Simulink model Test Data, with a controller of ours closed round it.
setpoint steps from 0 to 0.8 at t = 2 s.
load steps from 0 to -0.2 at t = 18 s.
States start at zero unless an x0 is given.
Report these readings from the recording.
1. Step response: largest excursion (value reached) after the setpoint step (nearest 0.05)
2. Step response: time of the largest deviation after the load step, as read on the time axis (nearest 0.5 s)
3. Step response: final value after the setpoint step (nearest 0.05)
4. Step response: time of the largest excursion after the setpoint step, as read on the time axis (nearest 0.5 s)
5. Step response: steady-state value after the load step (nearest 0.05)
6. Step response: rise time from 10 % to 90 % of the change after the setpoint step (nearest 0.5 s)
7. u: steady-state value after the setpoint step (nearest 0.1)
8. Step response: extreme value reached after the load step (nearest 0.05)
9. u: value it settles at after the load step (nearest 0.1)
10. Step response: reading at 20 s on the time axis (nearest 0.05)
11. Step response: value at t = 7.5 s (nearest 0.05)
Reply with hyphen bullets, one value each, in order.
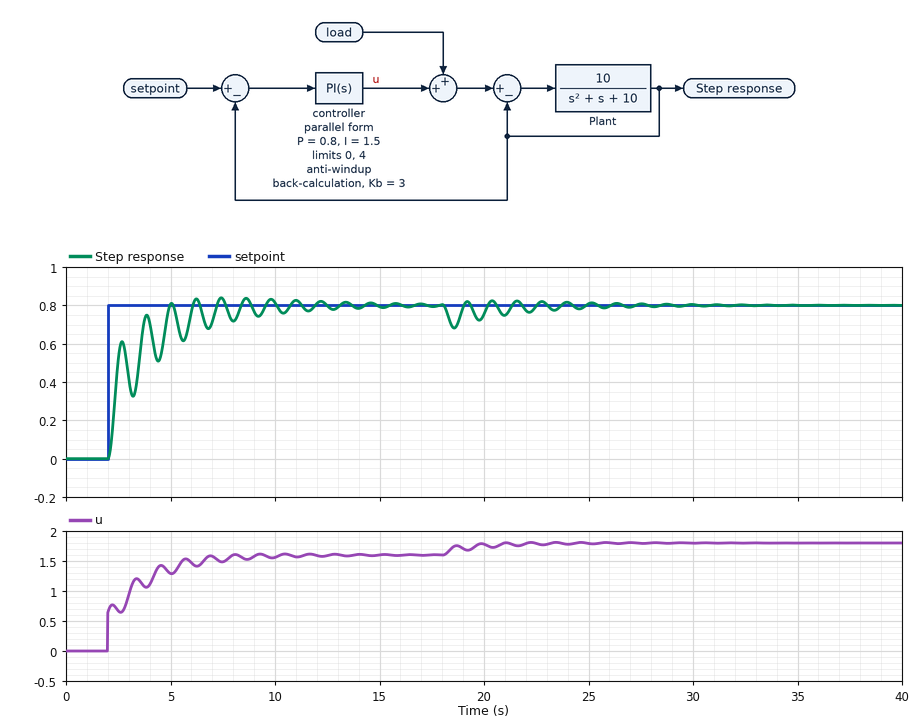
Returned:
- 0.85
- 18.5 s
- 0.80
- 7.5 s
- 0.80
- 1.5 s
- 1.6
- 0.70
- 1.8
- 0.75
- 0.85
